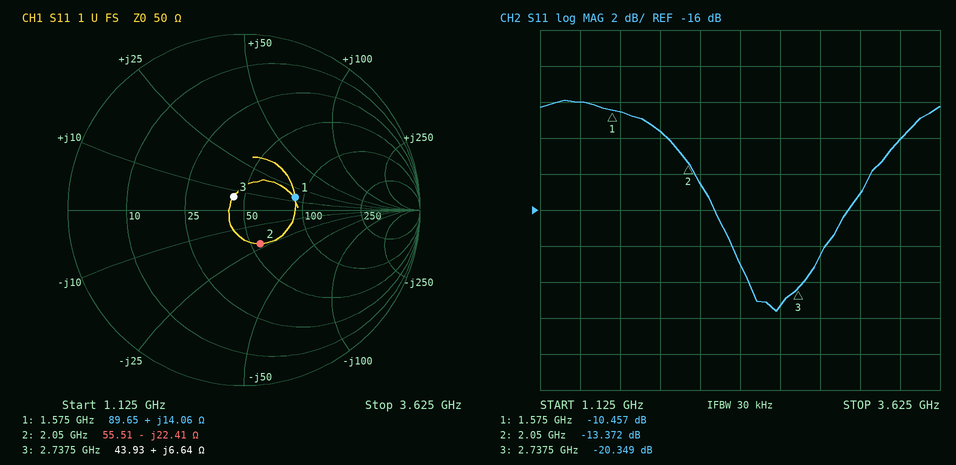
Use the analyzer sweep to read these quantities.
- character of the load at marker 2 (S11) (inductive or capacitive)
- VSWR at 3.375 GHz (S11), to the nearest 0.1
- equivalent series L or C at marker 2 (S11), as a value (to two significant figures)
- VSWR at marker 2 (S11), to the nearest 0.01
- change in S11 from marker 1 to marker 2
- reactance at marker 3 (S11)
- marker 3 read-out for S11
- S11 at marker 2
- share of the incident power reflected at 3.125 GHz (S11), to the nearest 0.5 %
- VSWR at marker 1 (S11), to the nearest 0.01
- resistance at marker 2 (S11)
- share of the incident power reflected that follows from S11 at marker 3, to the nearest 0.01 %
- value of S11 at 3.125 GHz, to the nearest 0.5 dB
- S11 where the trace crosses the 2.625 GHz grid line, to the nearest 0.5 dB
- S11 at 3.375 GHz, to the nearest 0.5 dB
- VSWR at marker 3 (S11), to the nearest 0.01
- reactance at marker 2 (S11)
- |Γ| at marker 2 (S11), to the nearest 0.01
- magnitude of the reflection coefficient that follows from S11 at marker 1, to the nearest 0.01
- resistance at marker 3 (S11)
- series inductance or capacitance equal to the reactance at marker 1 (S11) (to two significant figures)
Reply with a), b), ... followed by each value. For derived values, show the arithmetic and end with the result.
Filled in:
a) capacitive
b) |Γ| = 10^(-12/20) = 0.2512; VSWR = (1 + 0.2512)/(1 − 0.2512) ≈ 1.7
c) C = 1/(2π × 2.05 GHz × 22.41 Ω) ≈ 3.5 pF
d) (1 + 0.2145)/(1 − 0.2145) ≈ 1.55
e) -13.372 − (-10.457) = -2.915 dB
f) +6.64 Ω
g) -20.349 dB
h) -13.372 dB
i) 10^(-15/10) ≈ 3.16 %, so 3.0 % to the nearest 0.5 %
j) 1.86
k) 55.51 Ω
l) 10^(-20.349/10) ≈ 0.92 %
m) -15.0 dB
n) -21.5 dB
o) -12.0 dB
p) 1.21
q) -22.41 Ω
r) 0.21
s) 10^(-10.457/20) ≈ 0.30
t) 43.93 Ω
u) L = 14.06 Ω/(2π × 1.575 GHz) ≈ 1.4 nH
